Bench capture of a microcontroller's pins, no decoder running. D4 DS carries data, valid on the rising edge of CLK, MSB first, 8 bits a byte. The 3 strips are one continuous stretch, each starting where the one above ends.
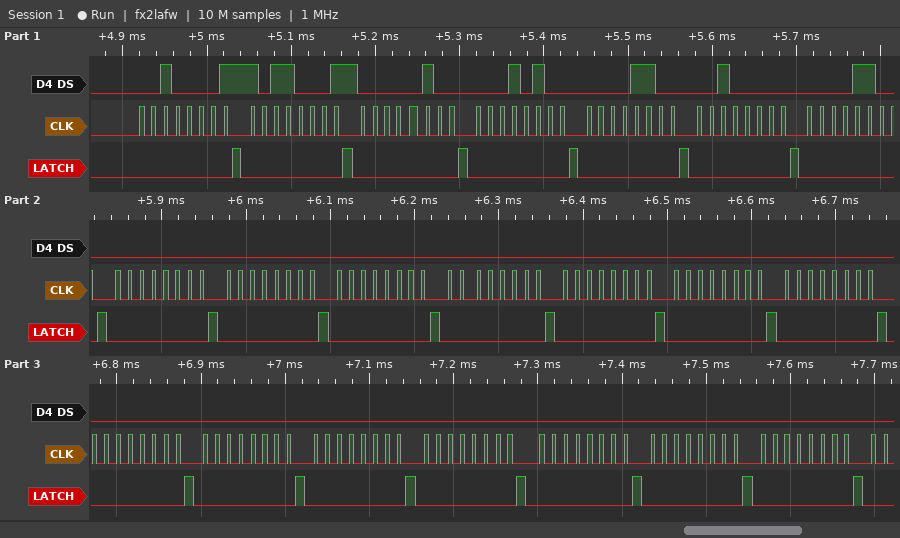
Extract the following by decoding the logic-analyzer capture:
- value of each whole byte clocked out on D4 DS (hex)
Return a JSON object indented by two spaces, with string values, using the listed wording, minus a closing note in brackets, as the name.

{
  "value of each whole byte clocked out on D4 DS": "21 B1 04 14 0C 20 0C 00 00 00 00 00 00 00 00 00 00 00 00 00 00"
}
